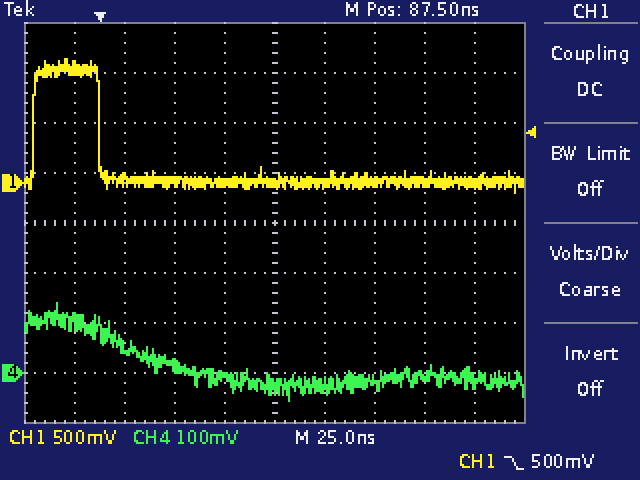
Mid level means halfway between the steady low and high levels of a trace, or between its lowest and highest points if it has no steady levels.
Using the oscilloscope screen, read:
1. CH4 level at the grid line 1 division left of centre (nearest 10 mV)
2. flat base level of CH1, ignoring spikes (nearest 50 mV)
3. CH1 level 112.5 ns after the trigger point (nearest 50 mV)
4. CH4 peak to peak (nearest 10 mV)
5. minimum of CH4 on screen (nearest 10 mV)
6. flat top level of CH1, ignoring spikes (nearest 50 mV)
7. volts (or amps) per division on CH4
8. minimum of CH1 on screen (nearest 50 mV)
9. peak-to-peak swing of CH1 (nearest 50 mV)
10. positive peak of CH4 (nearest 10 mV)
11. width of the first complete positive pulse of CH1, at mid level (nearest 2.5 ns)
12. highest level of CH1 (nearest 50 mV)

-10 mV
0 mV
0 mV
200 mV
-60 mV
1.15 V
100 mV
-100 mV
1.35 V
140 mV
32.5 ns
1.25 V
